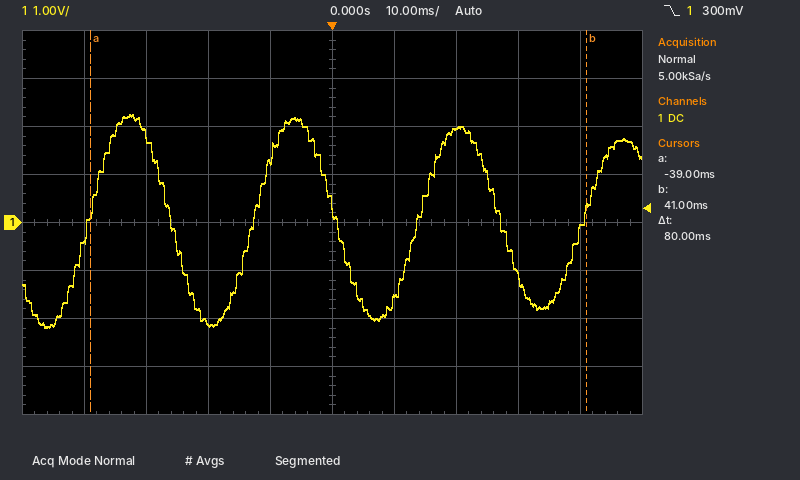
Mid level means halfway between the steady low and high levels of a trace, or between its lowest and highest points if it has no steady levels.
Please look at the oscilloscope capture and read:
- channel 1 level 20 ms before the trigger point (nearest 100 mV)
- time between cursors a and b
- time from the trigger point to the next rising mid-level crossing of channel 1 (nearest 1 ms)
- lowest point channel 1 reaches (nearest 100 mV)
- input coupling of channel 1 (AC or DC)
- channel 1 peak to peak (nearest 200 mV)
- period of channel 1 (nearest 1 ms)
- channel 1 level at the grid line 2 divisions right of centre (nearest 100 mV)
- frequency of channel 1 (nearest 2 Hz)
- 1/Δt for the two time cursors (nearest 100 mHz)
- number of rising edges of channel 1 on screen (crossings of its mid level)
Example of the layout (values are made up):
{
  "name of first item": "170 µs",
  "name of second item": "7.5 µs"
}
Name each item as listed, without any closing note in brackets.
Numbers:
{
  "channel 1 level 20 ms before the trigger point": "-2.1 V",
  "time between cursors a and b": "80 ms",
  "time from the trigger point to the next rising mid-level crossing of channel 1": "14 ms",
  "lowest point channel 1 reaches": "-2.2 V",
  "input coupling of channel 1": "DC",
  "channel 1 peak to peak": "4.4 V",
  "period of channel 1": "27 ms",
  "channel 1 level at the grid line 2 divisions right of centre": "2.0 V",
  "frequency of channel 1": "38 Hz",
  "1/Δt for the two time cursors": "12.5 Hz",
  "number of rising edges of channel 1 on screen": "4"
}
